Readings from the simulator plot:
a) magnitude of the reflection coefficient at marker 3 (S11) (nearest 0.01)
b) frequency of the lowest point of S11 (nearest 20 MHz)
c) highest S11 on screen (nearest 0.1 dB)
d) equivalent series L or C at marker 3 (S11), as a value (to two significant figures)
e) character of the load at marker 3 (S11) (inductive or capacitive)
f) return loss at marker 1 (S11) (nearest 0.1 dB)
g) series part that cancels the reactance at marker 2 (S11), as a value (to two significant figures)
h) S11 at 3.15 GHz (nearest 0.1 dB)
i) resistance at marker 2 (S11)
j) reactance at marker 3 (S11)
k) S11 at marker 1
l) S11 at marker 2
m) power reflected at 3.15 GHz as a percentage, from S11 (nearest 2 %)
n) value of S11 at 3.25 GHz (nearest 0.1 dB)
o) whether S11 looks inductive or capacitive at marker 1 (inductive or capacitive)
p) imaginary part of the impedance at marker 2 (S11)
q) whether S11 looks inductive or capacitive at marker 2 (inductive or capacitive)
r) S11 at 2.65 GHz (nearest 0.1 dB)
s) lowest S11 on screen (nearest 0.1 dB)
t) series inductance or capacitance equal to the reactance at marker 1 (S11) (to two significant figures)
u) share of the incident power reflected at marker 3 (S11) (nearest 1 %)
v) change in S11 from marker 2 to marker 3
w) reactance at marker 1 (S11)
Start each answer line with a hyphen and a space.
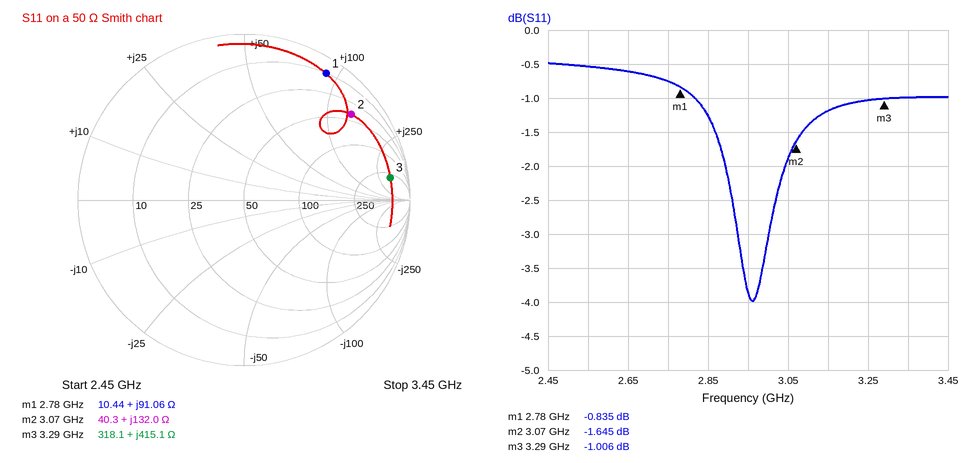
- 0.89
- 2.96 GHz
- -0.5 dB
- 20 nH
- inductive
- 0.8 dB
- 390 fF
- -1.2 dB
- 40.3 Ω
- +415.1 Ω
- -0.835 dB
- -1.645 dB
- 76 %
- -1.0 dB
- inductive
- +132.0 Ω
- inductive
- -0.6 dB
- -4.0 dB
- 5.2 nH
- 79 %
- 0.639 dB
- +91.06 Ω
